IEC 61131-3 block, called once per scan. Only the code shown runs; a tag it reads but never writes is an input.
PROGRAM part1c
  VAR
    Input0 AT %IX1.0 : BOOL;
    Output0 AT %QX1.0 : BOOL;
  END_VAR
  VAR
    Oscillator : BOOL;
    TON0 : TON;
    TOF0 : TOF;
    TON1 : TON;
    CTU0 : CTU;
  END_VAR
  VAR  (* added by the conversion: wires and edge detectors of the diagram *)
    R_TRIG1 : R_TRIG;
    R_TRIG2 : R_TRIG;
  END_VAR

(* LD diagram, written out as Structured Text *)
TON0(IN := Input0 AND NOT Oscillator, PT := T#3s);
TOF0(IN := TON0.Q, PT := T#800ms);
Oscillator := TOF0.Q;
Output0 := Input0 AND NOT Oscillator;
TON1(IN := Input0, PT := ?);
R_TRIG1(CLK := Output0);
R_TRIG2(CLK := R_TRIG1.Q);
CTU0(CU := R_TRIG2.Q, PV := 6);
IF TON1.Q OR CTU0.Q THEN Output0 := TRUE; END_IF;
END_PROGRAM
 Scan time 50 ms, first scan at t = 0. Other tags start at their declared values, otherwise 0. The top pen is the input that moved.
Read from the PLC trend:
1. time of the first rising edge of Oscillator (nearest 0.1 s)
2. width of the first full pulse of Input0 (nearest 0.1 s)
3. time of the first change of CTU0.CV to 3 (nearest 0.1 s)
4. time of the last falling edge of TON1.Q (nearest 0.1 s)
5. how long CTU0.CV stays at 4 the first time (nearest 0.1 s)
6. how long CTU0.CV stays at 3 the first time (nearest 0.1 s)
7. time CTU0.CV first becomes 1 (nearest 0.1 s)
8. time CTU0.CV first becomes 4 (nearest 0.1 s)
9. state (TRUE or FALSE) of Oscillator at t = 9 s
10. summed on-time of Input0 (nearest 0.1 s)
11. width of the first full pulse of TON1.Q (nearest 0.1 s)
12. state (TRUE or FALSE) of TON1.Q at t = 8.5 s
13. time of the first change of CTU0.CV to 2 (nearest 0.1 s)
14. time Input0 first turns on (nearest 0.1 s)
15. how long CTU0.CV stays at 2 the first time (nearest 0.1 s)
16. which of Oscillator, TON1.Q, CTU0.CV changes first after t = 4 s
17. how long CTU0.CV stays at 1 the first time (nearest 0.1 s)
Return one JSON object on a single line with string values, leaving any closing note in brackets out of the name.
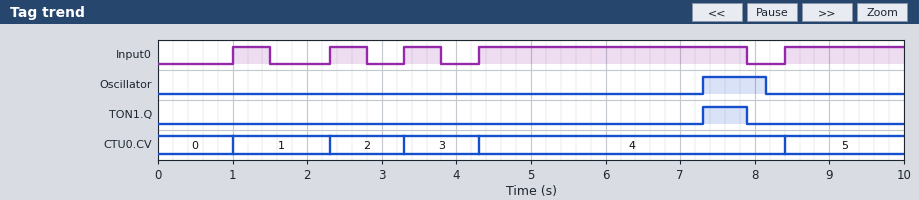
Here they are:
{"time of the first rising edge of Oscillator": "7.3 s", "width of the first full pulse of Input0": "0.5 s", "time of the first change of CTU0.CV to 3": "3.3 s", "time of the last falling edge of TON1.Q": "7.9 s", "how long CTU0.CV stays at 4 the first time": "4.1 s", "how long CTU0.CV stays at 3 the first time": "1.0 s", "time CTU0.CV first becomes 1": "1.0 s", "time CTU0.CV first becomes 4": "4.3 s", "state (TRUE or FALSE) of Oscillator at t = 9 s": "FALSE", "summed on-time of Input0": "6.7 s", "width of the first full pulse of TON1.Q": "0.6 s", "state (TRUE or FALSE) of TON1.Q at t = 8.5 s": "FALSE", "time of the first change of CTU0.CV to 2": "2.3 s", "time Input0 first turns on": "1.0 s", "how long CTU0.CV stays at 2 the first time": "1.0 s", "which of Oscillator, TON1.Q, CTU0.CV changes first after t = 4 s": "CTU0.CV", "how long CTU0.CV stays at 1 the first time": "1.3 s"}
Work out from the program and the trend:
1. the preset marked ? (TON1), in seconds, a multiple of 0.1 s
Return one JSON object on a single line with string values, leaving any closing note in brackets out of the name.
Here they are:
{"the preset marked ? (TON1), in seconds, a multiple of 0.1 s": "3.0 s"}
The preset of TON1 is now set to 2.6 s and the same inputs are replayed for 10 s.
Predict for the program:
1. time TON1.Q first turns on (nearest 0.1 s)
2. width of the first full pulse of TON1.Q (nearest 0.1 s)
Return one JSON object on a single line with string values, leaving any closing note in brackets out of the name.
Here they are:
{"time TON1.Q first turns on": "6.9 s", "width of the first full pulse of TON1.Q": "1.0 s"}
